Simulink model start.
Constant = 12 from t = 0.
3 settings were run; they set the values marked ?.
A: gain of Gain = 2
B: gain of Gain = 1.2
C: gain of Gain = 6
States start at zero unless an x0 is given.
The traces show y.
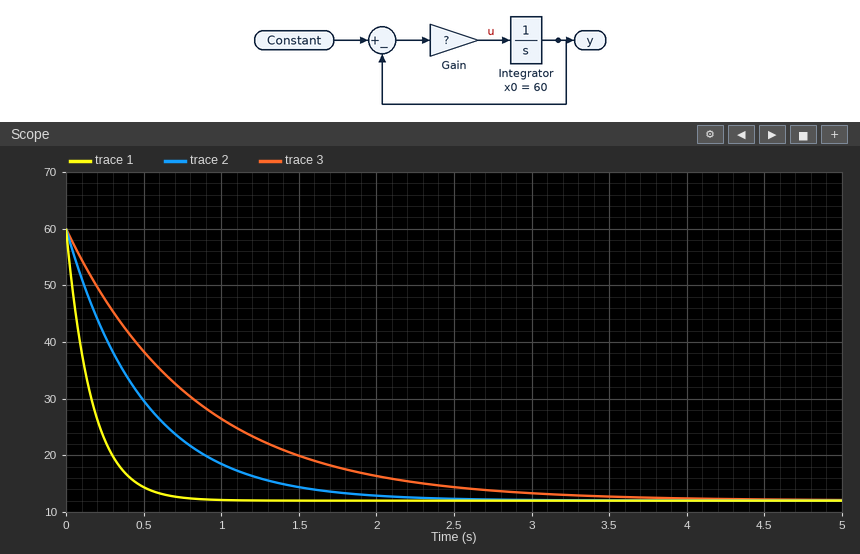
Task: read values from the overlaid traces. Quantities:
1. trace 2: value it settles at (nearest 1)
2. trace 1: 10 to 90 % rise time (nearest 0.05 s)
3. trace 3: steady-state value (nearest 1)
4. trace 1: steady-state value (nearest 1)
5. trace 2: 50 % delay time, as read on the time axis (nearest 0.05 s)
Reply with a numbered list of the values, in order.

1. 12
2. 0.35 s
3. 12
4. 12
5. 0.35 s
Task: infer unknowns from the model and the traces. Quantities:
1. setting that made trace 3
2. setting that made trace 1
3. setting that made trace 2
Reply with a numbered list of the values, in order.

1. B
2. C
3. A
